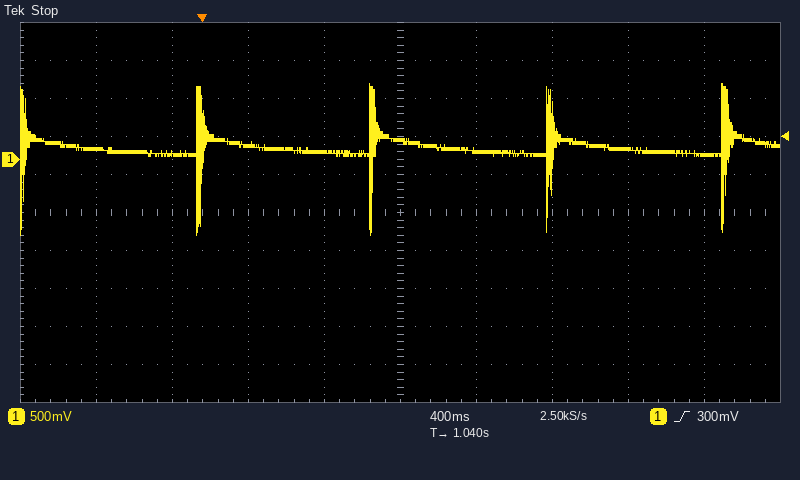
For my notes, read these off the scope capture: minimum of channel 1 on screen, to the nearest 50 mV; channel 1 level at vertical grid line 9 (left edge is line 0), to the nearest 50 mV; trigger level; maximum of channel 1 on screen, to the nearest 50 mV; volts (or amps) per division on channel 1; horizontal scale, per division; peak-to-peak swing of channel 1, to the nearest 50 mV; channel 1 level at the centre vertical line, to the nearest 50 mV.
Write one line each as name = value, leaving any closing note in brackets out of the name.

minimum of channel 1 on screen, to the nearest 50 mV = -1.00 V
channel 1 level at vertical grid line 9 (left edge is line 0), to the nearest 50 mV = 50 mV
trigger level = 300 mV
maximum of channel 1 on screen, to the nearest 50 mV = 1.00 V
volts (or amps) per division on channel 1 = 500 mV
horizontal scale, per division = 400 ms
peak-to-peak swing of channel 1, to the nearest 50 mV = 2.00 V
channel 1 level at the centre vertical line, to the nearest 50 mV = 250 mV
